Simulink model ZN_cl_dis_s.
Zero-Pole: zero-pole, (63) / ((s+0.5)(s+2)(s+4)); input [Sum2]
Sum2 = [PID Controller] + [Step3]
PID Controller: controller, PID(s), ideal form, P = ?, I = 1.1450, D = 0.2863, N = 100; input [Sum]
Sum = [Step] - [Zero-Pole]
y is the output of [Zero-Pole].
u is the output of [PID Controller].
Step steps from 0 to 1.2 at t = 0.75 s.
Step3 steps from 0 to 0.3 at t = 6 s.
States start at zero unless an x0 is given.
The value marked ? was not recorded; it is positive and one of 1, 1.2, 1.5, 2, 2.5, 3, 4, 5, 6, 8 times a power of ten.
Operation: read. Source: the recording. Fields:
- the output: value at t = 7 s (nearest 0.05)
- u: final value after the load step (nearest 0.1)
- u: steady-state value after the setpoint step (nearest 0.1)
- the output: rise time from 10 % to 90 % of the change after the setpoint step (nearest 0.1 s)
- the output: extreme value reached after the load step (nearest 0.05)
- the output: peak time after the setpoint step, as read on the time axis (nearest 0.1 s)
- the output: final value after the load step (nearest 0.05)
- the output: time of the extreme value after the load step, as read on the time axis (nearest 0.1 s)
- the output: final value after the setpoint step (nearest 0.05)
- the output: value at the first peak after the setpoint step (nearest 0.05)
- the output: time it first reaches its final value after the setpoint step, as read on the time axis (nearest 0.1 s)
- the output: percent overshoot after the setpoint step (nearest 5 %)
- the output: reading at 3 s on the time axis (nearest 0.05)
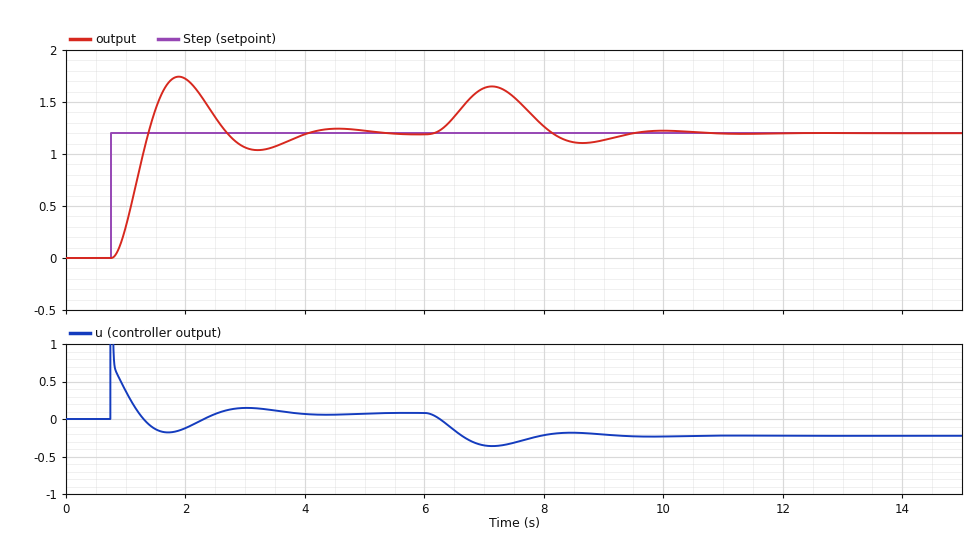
1.65
-0.2
0.1
0.4 s
1.65
1.9 s
1.20
7.1 s
1.20
1.75
1.4 s
45 %
1.05
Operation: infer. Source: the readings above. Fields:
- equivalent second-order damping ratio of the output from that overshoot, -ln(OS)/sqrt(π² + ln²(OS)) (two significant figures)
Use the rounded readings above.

0.25
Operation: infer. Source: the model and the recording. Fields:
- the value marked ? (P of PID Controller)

0.6
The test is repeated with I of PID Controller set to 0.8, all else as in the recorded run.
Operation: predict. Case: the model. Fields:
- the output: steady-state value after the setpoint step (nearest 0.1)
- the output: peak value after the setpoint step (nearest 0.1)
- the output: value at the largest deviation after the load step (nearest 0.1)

1.2
1.6
1.7
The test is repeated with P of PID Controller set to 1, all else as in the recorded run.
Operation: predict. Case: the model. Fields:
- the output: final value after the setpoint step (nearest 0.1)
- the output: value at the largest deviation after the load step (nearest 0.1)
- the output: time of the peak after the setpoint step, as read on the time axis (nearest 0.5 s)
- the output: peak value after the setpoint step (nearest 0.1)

1.2
1.5
1.5 s
1.8
